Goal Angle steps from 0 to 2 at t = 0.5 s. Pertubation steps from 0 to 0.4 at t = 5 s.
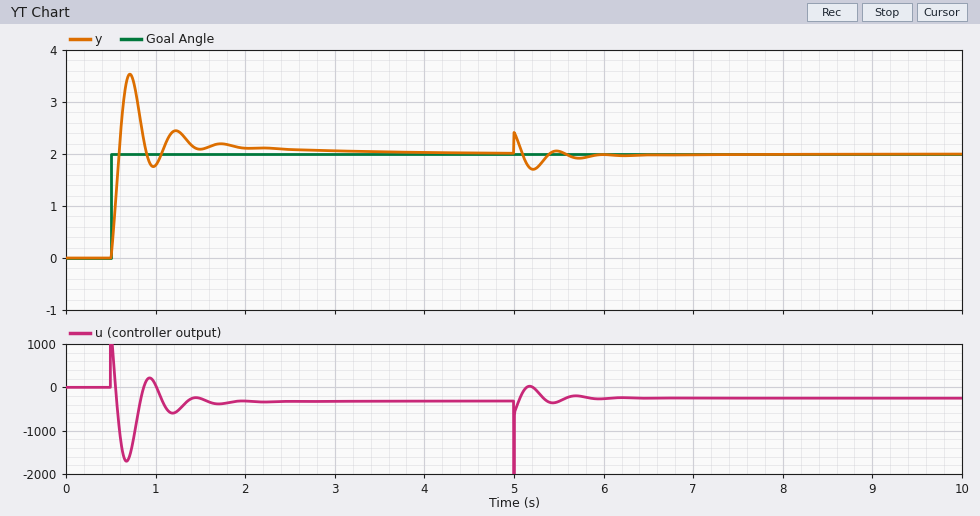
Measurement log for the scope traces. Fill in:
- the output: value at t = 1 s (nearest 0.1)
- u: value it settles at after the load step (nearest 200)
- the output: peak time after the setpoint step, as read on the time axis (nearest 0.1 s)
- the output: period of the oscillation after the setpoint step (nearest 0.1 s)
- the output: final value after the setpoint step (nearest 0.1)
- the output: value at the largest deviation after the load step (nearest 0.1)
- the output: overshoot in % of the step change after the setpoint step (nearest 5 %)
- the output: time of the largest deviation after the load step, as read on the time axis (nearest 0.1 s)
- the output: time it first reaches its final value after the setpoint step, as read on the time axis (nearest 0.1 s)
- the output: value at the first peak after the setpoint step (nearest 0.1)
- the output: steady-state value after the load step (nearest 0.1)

1.8
-200
0.7 s
0.5 s
2.0
2.4
75 %
5.0 s
0.6 s
3.5
2.0
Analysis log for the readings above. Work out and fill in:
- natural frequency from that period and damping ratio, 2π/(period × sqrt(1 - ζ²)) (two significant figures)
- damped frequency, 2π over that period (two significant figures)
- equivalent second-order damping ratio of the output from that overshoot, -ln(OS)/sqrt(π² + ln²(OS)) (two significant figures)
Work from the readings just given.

13 rad/s
13 rad/s
0.091
